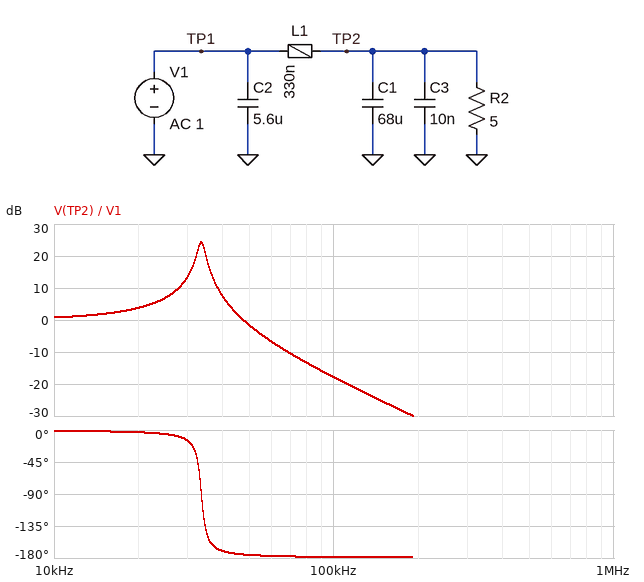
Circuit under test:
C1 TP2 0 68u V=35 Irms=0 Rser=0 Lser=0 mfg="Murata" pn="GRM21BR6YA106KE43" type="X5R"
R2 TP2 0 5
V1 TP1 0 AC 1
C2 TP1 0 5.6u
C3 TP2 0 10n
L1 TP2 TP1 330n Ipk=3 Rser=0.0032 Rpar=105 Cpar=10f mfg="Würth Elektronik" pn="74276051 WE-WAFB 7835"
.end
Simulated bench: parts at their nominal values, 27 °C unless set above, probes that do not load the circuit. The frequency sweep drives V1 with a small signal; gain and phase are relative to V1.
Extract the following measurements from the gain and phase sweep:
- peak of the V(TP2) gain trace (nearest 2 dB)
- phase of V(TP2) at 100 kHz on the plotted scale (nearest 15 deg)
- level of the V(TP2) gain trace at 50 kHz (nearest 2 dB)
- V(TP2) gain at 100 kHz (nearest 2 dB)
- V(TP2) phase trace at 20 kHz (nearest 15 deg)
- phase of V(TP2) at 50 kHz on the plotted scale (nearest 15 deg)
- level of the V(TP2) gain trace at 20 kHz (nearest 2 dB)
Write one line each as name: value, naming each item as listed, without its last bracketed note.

peak of the V(TP2) gain trace: 24 dB
phase of V(TP2) at 100 kHz on the plotted scale: -180 deg
level of the V(TP2) gain trace at 50 kHz: -2 dB
V(TP2) gain at 100 kHz: -18 dB
V(TP2) phase trace at 20 kHz: 0 deg
phase of V(TP2) at 50 kHz on the plotted scale: -180 deg
level of the V(TP2) gain trace at 20 kHz: 4 dB
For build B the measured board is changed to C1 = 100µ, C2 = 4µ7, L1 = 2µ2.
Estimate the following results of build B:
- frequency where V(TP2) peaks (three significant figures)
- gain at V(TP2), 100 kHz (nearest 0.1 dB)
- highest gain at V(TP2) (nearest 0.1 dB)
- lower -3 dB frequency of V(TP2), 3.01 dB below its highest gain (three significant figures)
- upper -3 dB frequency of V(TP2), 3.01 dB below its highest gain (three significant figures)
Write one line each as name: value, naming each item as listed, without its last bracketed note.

frequency where V(TP2) peaks: 10.7 kHz
gain at V(TP2), 100 kHz: -38.7 dB
highest gain at V(TP2): 25.6 dB
lower -3 dB frequency of V(TP2), 3.01 dB below its highest gain: 10.4 kHz
upper -3 dB frequency of V(TP2), 3.01 dB below its highest gain: 11.0 kHz
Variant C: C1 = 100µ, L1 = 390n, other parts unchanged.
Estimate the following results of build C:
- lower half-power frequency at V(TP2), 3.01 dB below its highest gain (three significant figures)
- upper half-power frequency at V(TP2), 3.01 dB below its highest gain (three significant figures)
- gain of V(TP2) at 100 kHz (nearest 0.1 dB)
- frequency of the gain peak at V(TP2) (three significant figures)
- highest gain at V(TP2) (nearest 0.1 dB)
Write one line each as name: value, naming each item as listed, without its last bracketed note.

lower half-power frequency at V(TP2), 3.01 dB below its highest gain: 24.6 kHz
upper half-power frequency at V(TP2), 3.01 dB below its highest gain: 26.3 kHz
gain of V(TP2) at 100 kHz: -23.2 dB
frequency of the gain peak at V(TP2): 25.5 kHz
highest gain at V(TP2): 23.8 dB
